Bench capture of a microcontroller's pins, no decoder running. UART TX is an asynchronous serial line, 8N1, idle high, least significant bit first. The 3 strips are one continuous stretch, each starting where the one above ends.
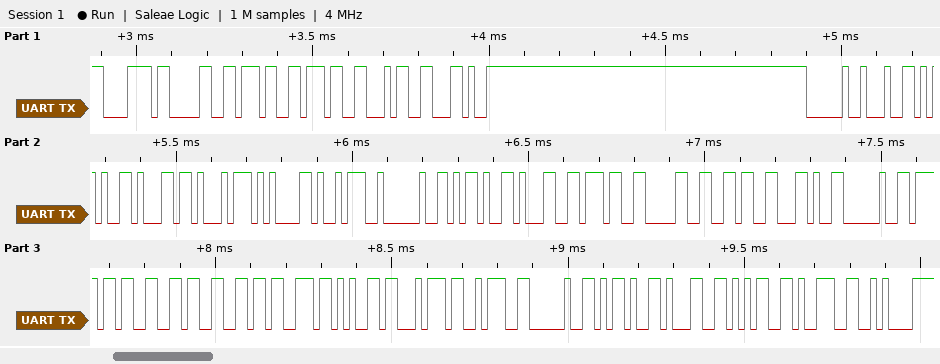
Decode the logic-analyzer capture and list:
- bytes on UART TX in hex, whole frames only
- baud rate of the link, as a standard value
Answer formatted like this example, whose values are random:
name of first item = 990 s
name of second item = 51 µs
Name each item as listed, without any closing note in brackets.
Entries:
bytes on UART TX in hex, whole frames only = 78 30 37 37 34 2C 20 64 65 6C 74 61 3A 20 2D 31 37 30 36 2C 20 6F 66 66 73 65 74 3A 20 2D 31 35 39 0A
baud rate of the link, as a standard value = 57600 baud
